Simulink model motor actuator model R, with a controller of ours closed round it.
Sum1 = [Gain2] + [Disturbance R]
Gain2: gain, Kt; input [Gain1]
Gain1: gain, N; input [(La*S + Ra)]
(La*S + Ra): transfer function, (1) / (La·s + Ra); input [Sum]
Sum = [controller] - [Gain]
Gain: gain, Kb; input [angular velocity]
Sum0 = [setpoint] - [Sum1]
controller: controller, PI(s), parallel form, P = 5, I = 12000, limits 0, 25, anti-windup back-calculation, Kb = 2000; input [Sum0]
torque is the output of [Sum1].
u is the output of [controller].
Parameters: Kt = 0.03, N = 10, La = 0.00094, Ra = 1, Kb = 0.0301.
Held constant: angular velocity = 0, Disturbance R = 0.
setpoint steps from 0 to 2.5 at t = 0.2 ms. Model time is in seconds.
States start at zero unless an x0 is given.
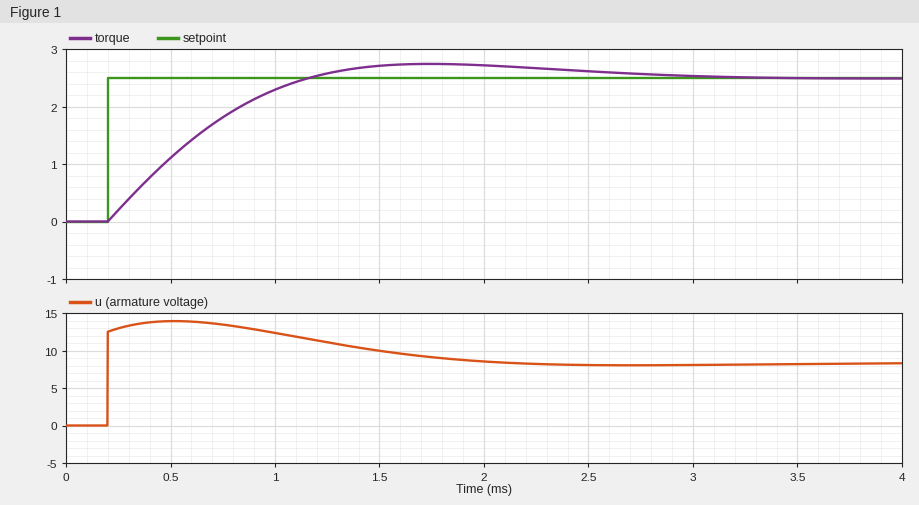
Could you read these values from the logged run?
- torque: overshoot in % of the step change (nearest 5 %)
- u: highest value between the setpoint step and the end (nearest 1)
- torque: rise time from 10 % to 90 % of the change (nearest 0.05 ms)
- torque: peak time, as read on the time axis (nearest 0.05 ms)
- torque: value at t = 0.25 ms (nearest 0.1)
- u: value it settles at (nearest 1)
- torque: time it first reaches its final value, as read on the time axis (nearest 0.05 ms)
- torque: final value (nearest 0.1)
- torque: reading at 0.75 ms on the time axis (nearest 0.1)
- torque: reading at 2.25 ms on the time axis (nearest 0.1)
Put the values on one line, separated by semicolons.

10 %; 14; 0.70 ms; 1.75 ms; 0.2; 8; 1.15 ms; 2.5; 1.8; 2.7
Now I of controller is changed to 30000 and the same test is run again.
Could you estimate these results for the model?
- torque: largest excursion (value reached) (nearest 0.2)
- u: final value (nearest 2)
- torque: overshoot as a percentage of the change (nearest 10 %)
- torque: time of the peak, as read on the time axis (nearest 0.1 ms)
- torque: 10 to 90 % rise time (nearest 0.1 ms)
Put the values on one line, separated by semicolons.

3.2; 8; 30 %; 1.1 ms; 0.4 ms
